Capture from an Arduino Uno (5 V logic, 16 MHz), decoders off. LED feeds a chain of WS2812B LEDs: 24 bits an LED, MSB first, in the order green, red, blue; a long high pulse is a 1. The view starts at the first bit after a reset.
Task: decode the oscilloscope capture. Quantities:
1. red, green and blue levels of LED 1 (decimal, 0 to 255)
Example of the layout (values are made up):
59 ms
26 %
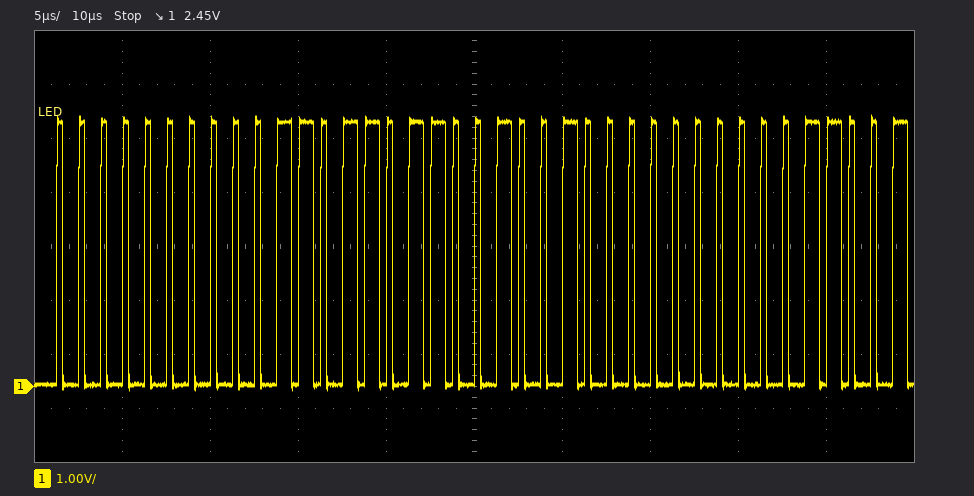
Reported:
54, 0, 201
